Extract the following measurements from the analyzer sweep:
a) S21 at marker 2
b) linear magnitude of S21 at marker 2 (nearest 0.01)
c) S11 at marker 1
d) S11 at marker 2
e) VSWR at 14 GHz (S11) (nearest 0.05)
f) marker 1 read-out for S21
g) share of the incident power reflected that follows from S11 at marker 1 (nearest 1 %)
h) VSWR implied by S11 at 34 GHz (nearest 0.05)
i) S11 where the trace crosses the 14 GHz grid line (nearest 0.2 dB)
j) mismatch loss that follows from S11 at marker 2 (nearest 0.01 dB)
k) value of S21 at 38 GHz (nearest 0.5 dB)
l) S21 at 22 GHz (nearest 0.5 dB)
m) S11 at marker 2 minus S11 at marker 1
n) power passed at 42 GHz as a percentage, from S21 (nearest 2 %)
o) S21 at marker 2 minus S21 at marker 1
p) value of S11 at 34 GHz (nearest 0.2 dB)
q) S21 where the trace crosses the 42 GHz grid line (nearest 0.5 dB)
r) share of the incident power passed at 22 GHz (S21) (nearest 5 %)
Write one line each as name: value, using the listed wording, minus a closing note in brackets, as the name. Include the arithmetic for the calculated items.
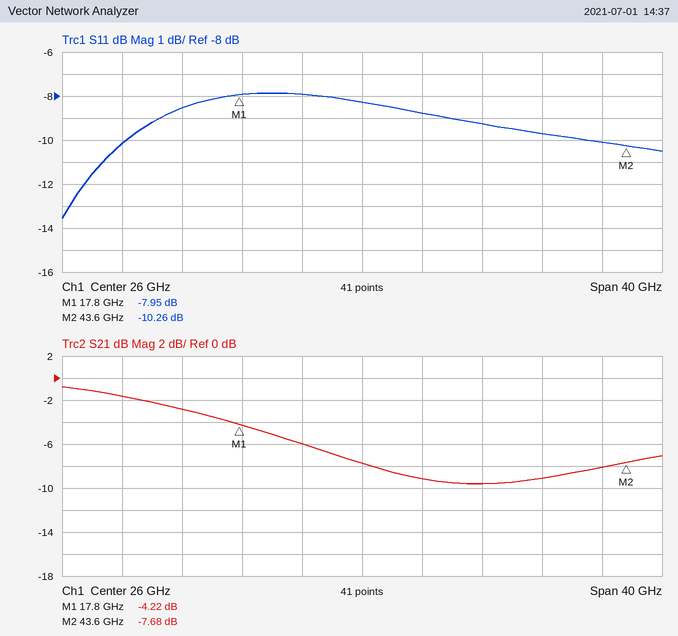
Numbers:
S21 at marker 2: -7.68 dB
linear magnitude of S21 at marker 2: 10^(-7.68/20) ≈ 0.41
S11 at marker 1: -7.95 dB
S11 at marker 2: -10.26 dB
VSWR at 14 GHz (S11): |Γ| = 10^(-8.6/20) = 0.3715; VSWR = (1 + 0.3715)/(1 − 0.3715) ≈ 2.18, so 2.20 to the nearest 0.05
marker 1 read-out for S21: -4.22 dB
share of the incident power reflected that follows from S11 at marker 1: 10^(-7.95/10) ≈ 16 %
VSWR implied by S11 at 34 GHz: |Γ| = 10^(-9.2/20) = 0.3467; VSWR = (1 + 0.3467)/(1 − 0.3467) ≈ 2.06, so 2.05 to the nearest 0.05
S11 where the trace crosses the 14 GHz grid line: -8.6 dB
mismatch loss that follows from S11 at marker 2: −10 log10(1 − 10^(-10.26/10)) ≈ 0.43 dB
value of S21 at 38 GHz: -9.0 dB
S21 at 22 GHz: -6.0 dB
S11 at marker 2 minus S11 at marker 1: -10.26 − (-7.95) = -2.31 dB
power passed at 42 GHz as a percentage, from S21: 10^(-8/10) ≈ 16 %
S21 at marker 2 minus S21 at marker 1: -7.68 − (-4.22) = -3.46 dB
value of S11 at 34 GHz: -9.2 dB
S21 where the trace crosses the 42 GHz grid line: -8.0 dB
share of the incident power passed at 22 GHz (S21): 10^(-6/10) ≈ 25 %
